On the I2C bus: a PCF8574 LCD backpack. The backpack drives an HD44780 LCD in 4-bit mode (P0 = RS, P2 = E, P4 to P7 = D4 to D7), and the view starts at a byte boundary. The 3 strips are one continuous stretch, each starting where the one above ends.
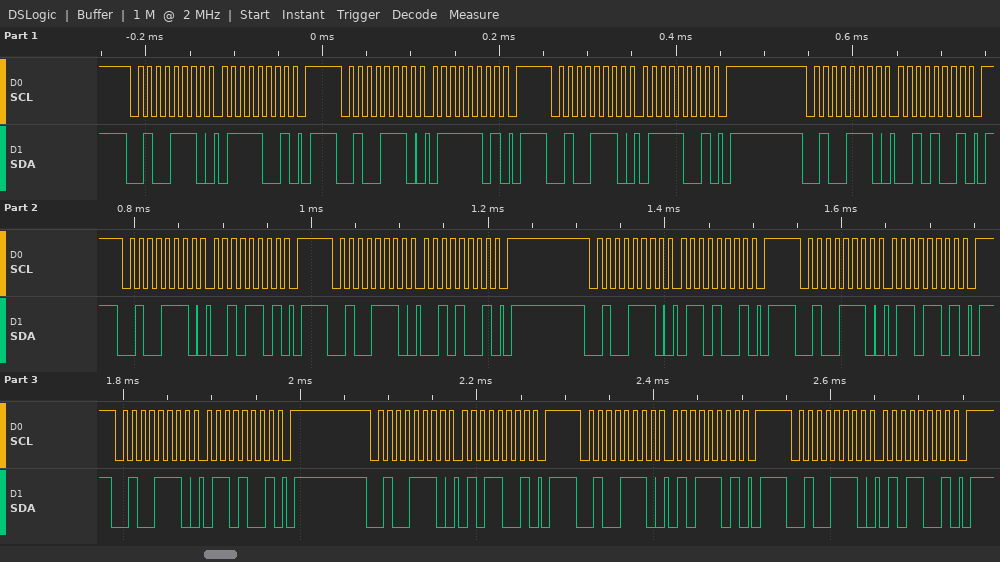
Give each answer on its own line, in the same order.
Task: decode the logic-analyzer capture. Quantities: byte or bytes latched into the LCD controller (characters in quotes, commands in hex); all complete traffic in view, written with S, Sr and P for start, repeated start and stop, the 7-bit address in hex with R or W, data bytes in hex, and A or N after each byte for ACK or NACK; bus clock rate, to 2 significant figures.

'r' 'e'
S 27W A 79 A P S 27W A 7D A P S 27W A 79 A P S 27W A 29 A P S 27W A 2D A P S 27W A 29 A P S 27W A 69 A P S 27W A 6D A P S 27W A 69 A P S 27W A 59 A P S 27W A 5D A P S 27W A 59 A P
100 kHz
